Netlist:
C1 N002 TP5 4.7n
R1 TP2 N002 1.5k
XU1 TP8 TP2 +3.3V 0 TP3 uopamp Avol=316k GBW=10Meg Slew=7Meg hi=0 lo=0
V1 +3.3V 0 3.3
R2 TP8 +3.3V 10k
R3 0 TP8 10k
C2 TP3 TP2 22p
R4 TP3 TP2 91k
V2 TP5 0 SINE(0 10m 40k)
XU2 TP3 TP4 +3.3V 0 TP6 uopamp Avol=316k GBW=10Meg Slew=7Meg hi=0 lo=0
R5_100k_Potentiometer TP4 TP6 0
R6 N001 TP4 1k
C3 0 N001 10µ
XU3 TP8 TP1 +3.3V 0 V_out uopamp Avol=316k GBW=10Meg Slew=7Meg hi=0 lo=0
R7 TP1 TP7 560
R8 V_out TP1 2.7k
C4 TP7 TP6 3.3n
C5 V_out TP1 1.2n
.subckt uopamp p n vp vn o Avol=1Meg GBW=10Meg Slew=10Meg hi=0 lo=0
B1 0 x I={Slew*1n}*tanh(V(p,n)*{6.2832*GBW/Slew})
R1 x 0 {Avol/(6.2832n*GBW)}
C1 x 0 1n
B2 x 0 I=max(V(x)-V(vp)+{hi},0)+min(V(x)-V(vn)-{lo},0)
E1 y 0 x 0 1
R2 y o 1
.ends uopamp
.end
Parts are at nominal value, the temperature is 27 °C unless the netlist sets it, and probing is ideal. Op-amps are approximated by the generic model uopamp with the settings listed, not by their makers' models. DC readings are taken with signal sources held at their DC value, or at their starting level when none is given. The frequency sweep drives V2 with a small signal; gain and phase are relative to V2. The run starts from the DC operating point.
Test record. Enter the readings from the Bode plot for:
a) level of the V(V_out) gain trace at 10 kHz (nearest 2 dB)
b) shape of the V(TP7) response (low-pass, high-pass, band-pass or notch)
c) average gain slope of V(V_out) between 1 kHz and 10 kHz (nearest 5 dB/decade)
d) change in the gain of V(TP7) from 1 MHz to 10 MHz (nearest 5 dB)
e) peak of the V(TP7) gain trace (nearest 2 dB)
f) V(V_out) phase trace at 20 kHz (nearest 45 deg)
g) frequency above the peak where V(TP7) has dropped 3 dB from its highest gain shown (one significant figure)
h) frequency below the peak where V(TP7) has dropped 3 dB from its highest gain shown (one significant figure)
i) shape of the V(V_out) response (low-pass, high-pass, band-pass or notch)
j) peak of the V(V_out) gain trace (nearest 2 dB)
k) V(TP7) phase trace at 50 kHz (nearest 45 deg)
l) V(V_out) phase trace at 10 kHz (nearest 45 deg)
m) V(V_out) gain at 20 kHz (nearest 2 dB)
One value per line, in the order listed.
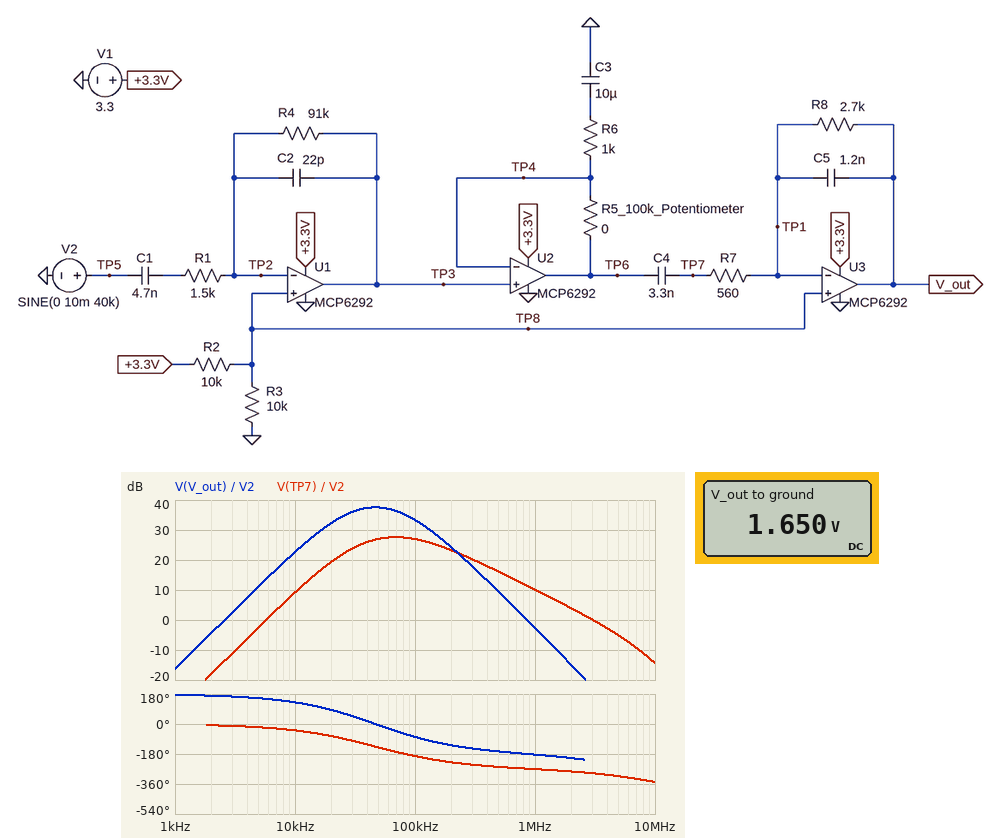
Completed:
22 dB
band-pass
40 dB/decade
-25 dB
28 dB
90 deg
200 kHz
30 kHz
band-pass
38 dB
-135 deg
135 deg
32 dB
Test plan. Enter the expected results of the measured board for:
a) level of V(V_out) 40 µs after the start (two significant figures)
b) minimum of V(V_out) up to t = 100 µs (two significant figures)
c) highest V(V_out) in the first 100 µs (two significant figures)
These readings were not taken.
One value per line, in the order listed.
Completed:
1.1 V
910 mV
2.4 V
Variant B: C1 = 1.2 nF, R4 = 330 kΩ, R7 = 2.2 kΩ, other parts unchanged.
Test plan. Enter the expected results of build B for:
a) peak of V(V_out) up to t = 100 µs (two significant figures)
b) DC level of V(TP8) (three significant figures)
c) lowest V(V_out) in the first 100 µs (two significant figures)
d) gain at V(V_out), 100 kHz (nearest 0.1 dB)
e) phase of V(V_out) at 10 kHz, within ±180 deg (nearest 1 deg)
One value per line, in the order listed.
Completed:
2.0 V
1.65 V
1.3 V
23.5 dB
112 deg
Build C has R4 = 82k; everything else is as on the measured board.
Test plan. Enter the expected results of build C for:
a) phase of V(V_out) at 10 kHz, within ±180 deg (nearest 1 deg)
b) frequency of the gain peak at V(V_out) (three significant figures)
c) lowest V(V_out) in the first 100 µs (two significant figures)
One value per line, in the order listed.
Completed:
131 deg
48.4 kHz
970 mV
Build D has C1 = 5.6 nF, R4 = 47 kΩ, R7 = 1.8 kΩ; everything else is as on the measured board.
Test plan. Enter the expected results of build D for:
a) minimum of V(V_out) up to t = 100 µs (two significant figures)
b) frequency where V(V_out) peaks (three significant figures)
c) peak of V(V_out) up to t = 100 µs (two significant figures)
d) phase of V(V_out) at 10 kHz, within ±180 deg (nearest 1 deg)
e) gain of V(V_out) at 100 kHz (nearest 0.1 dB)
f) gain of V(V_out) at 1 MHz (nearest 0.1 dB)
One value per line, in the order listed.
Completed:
1.4 V
39.1 kHz
1.9 V
116 deg
23.3 dB
-12.7 dB
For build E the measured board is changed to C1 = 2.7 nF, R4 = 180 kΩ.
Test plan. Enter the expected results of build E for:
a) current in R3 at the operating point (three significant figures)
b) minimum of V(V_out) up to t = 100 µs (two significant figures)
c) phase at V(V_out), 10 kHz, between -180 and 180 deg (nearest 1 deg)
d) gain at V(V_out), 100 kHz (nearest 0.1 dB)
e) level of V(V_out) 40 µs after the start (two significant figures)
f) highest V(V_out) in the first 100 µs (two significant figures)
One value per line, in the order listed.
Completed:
165 µA
720 mV
133 deg
34.0 dB
970 mV
2.6 V
